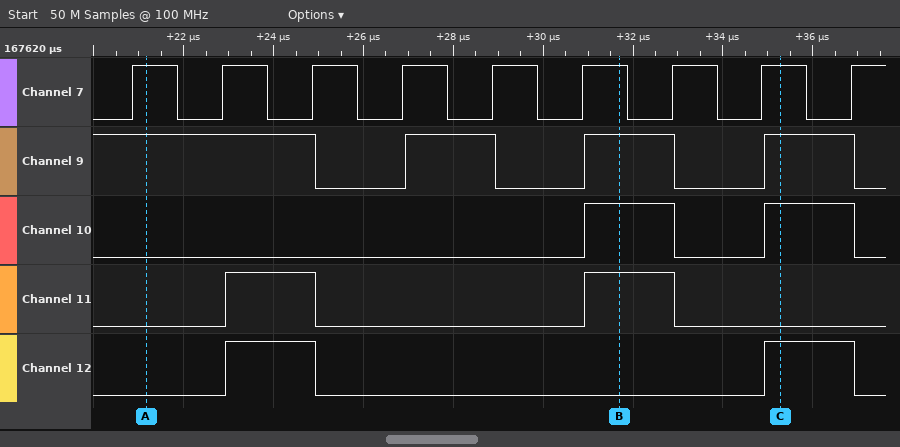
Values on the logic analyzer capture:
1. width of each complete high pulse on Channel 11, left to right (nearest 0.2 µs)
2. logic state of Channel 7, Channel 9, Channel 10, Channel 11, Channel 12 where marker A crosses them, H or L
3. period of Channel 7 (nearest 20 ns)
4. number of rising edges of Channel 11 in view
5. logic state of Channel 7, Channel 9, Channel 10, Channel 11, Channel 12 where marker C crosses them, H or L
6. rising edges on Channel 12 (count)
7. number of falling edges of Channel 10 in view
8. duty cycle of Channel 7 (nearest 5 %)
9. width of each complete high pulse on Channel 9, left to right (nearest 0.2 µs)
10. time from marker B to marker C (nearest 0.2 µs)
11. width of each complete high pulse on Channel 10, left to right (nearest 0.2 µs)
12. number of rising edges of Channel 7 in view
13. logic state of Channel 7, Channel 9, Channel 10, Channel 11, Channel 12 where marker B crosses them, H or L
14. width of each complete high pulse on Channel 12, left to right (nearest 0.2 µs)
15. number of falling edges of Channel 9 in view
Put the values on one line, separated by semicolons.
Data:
2 µs, 2 µs; Channel 7=H, Channel 9=H, Channel 10=L, Channel 11=L, Channel 12=L; 2000 ns; 2; Channel 7=H, Channel 9=H, Channel 10=H, Channel 11=L, Channel 12=H; 2; 2; 50 %; 2 µs, 2 µs, 2 µs; 3.6 µs; 2 µs, 2 µs; 9; Channel 7=H, Channel 9=H, Channel 10=H, Channel 11=H, Channel 12=L; 2 µs, 2 µs; 4
